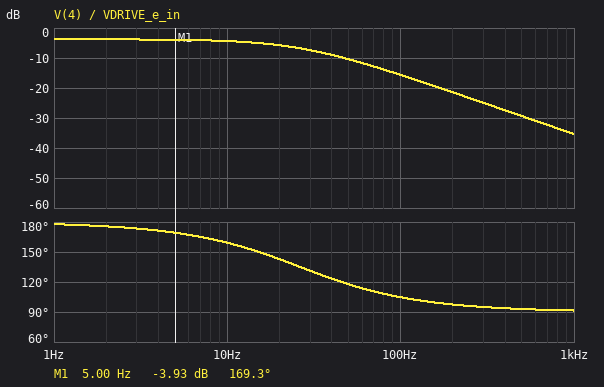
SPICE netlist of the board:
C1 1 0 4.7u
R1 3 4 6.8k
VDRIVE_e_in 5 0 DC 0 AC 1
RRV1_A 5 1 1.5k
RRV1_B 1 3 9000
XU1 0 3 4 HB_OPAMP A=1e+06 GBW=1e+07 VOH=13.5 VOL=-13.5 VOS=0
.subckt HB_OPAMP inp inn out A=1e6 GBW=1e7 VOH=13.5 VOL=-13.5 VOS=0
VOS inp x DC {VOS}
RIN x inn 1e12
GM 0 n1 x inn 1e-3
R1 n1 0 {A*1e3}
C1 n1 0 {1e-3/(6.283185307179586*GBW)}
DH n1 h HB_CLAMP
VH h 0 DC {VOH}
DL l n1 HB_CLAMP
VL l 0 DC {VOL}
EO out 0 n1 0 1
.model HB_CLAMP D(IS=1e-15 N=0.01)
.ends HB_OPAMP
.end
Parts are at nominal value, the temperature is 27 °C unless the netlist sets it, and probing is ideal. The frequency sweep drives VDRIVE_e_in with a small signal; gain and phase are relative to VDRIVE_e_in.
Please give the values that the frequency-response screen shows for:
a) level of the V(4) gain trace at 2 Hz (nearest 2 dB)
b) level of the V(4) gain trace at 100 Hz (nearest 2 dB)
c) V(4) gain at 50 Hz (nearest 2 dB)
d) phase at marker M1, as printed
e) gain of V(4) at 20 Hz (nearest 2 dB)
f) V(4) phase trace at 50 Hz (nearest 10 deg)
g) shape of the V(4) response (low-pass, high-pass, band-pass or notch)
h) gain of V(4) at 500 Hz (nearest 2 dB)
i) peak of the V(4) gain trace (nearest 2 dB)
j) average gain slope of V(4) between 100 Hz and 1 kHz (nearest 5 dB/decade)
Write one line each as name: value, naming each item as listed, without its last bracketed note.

level of the V(4) gain trace at 2 Hz: -4 dB
level of the V(4) gain trace at 100 Hz: -16 dB
V(4) gain at 50 Hz: -10 dB
phase at marker M1, as printed: 169.3 deg
gain of V(4) at 20 Hz: -6 dB
V(4) phase trace at 50 Hz: 120 deg
shape of the V(4) response: low-pass
gain of V(4) at 500 Hz: -30 dB
peak of the V(4) gain trace: -4 dB
average gain slope of V(4) between 100 Hz and 1 kHz: -20 dB/decade
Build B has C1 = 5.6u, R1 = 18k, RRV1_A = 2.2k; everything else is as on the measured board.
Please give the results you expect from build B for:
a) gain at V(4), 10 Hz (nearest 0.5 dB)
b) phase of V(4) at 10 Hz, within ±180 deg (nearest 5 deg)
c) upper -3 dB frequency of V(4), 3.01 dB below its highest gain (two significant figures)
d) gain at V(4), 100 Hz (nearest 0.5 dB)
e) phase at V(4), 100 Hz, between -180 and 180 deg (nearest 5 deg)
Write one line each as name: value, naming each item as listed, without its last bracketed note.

gain at V(4), 10 Hz: 2.5 dB
phase of V(4) at 10 Hz, within ±180 deg: 150 deg
upper -3 dB frequency of V(4), 3.01 dB below its highest gain: 16 Hz
gain at V(4), 100 Hz: -12.0 dB
phase at V(4), 100 Hz, between -180 and 180 deg: 100 deg
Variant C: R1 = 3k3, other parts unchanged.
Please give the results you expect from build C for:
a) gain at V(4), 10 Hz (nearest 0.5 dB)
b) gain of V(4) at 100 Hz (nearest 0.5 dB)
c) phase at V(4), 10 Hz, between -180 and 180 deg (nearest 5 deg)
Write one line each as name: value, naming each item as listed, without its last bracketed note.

gain at V(4), 10 Hz: -10.5 dB
gain of V(4) at 100 Hz: -22.0 dB
phase at V(4), 10 Hz, between -180 and 180 deg: 160 deg
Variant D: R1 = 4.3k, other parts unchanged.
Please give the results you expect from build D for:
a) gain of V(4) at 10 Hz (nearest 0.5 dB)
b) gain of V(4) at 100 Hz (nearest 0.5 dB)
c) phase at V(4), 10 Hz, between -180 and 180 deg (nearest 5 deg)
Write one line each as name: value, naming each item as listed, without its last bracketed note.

gain of V(4) at 10 Hz: -8.5 dB
gain of V(4) at 100 Hz: -19.5 dB
phase at V(4), 10 Hz, between -180 and 180 deg: 160 deg
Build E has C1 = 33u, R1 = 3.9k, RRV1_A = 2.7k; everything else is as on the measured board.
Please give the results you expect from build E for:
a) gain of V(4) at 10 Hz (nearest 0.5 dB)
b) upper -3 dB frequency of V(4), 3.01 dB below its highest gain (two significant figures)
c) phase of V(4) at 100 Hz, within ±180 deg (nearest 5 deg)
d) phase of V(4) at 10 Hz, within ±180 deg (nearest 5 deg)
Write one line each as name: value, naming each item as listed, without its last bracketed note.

gain of V(4) at 10 Hz: -22.5 dB
upper -3 dB frequency of V(4), 3.01 dB below its highest gain: 2.3 Hz
phase of V(4) at 100 Hz, within ±180 deg: 90 deg
phase of V(4) at 10 Hz, within ±180 deg: 105 deg
